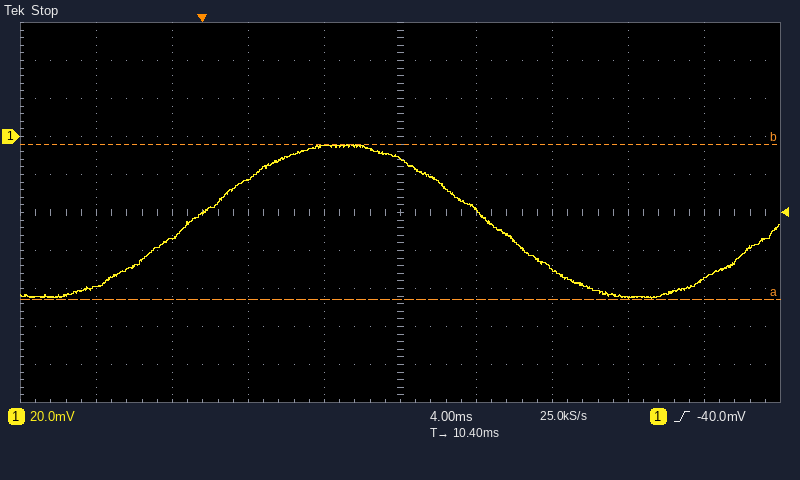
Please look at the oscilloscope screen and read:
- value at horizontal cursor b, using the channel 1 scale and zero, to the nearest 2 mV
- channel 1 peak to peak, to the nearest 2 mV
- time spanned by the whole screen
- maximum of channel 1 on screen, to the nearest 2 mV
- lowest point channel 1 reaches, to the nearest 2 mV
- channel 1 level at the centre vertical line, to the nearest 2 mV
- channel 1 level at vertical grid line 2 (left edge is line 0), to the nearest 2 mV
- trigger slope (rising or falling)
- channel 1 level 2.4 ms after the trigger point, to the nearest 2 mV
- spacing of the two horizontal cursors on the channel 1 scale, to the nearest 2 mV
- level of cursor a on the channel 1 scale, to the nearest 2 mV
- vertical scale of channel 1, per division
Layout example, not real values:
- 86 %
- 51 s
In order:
- -4 mV
- 82 mV
- 40 ms
- -4 mV
- -86 mV
- -12 mV
- -54 mV
- rising
- -22 mV
- 82 mV
- -86 mV
- 20 mV
